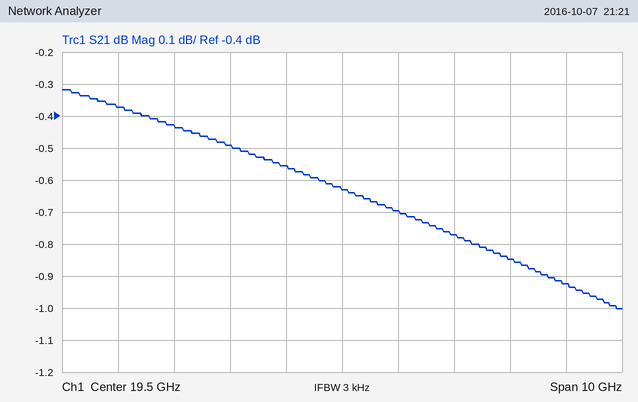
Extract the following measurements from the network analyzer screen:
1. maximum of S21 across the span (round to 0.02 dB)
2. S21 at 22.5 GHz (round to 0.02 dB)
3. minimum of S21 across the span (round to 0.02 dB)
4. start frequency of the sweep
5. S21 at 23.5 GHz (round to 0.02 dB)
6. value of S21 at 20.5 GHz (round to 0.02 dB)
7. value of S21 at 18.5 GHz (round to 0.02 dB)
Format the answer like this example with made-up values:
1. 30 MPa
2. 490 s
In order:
1. -0.32 dB
2. -0.84 dB
3. -1.00 dB
4. 14.5 GHz
5. -0.92 dB
6. -0.70 dB
7. -0.56 dB
